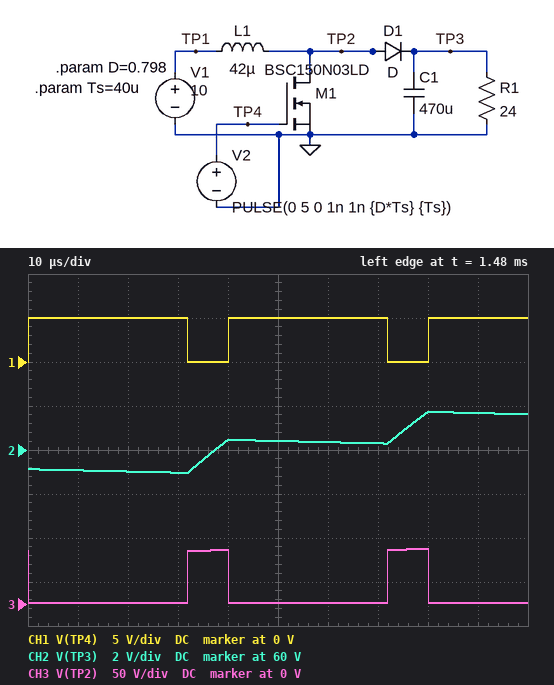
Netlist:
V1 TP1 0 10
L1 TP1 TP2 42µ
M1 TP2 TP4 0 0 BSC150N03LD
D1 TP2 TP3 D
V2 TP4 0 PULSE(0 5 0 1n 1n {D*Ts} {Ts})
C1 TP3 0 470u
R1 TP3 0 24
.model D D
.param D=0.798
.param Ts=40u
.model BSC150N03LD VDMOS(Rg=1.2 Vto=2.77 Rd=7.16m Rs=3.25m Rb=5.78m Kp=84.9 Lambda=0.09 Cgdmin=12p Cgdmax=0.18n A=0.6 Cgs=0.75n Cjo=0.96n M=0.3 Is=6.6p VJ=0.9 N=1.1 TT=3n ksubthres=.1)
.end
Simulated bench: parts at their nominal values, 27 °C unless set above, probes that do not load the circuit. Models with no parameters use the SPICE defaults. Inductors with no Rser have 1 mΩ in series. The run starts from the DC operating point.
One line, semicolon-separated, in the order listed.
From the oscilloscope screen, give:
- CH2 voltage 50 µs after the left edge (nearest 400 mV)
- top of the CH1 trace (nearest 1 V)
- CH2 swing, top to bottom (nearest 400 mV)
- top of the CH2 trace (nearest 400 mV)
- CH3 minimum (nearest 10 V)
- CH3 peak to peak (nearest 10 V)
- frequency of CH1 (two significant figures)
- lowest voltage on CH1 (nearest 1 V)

60.4 V; 5 V; 2.8 V; 61.6 V; 0 V; 60 V; 25 kHz; 0 V
